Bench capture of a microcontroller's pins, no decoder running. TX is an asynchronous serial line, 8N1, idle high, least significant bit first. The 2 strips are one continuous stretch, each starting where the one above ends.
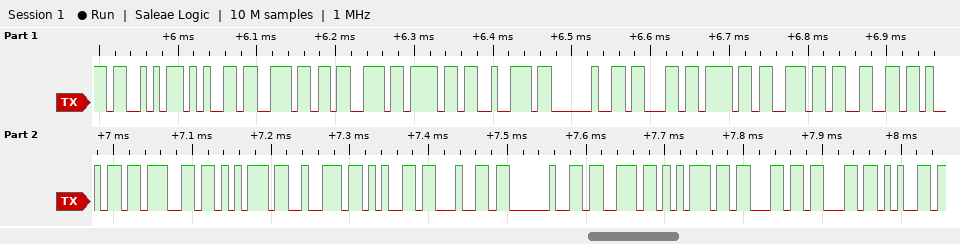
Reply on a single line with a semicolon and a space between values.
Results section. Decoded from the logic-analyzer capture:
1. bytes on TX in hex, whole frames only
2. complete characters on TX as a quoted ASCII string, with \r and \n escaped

53 65 6E 73 6F 72 20 63 6F 6E 66 69 67 75 72 65 64 20 73 75 63 63 65; "Sensor configured succe"
